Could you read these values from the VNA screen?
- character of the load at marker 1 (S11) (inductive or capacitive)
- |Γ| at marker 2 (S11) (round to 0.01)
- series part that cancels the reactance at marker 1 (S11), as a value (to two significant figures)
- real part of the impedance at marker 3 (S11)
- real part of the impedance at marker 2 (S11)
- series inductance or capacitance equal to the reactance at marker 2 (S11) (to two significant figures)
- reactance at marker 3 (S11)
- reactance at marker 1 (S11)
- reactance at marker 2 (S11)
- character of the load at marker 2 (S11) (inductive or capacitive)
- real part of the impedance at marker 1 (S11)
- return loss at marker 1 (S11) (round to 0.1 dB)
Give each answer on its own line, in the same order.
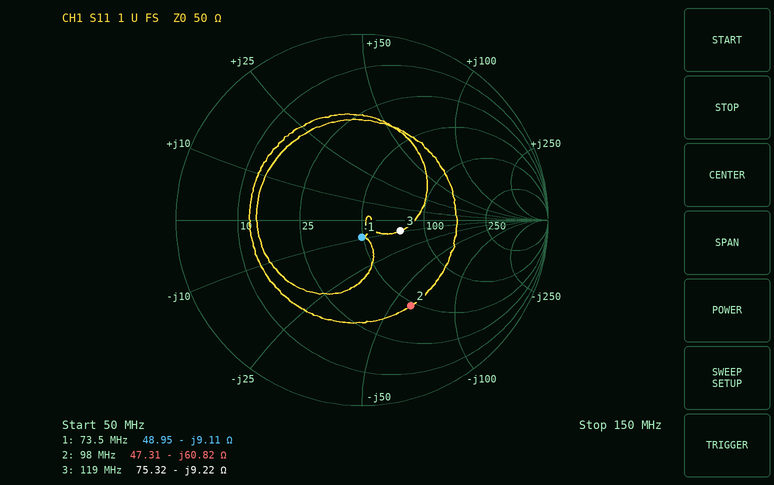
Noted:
capacitive
0.53
20 nH
75.32 Ω
47.31 Ω
27 pF
-9.22 Ω
-9.11 Ω
-60.82 Ω
capacitive
48.95 Ω
20.7 dB
